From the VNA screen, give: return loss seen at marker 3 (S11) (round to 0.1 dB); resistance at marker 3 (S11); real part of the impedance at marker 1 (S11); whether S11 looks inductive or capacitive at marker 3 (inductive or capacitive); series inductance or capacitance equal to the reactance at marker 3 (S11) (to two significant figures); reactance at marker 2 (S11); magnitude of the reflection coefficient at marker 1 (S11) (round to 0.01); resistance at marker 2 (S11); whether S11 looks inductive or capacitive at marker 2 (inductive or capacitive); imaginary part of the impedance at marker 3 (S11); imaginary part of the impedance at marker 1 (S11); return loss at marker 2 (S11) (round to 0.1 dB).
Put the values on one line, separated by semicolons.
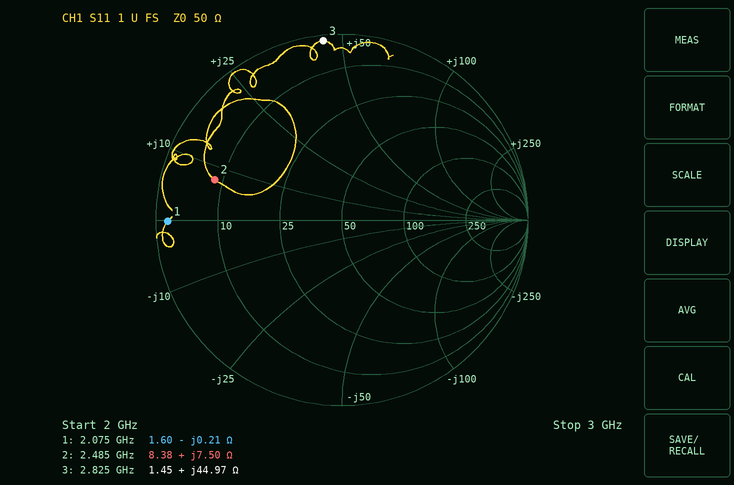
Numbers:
0.3 dB; 1.45 Ω; 1.60 Ω; inductive; 2.5 nH; +7.50 Ω; 0.94; 8.38 Ω; inductive; +44.97 Ω; -0.21 Ω; 2.9 dB
